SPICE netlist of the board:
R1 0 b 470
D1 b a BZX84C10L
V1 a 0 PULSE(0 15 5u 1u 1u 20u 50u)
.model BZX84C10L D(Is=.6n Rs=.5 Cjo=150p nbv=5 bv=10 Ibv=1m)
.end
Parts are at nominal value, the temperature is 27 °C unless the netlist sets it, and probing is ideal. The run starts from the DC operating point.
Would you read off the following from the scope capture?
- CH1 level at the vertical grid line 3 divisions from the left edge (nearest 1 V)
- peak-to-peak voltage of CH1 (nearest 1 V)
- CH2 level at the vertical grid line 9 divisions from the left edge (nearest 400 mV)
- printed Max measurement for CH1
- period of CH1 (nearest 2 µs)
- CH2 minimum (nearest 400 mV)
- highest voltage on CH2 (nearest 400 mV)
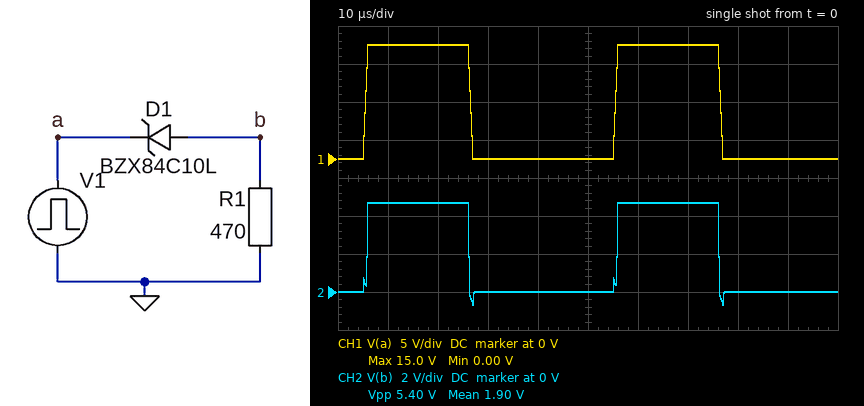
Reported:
0 V
15 V
0 V
15.0 V
50 µs
-800 mV
4.8 V
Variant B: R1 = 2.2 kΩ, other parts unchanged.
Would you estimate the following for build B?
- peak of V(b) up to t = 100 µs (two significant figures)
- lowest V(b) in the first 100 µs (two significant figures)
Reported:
4.9 V
-2.2 V
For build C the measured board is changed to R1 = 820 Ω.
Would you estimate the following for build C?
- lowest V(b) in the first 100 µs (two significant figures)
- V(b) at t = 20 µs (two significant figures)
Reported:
-1.1 V
4.8 V
